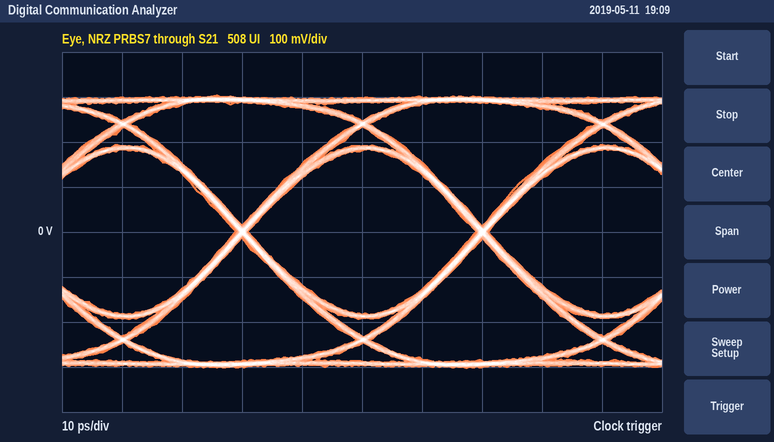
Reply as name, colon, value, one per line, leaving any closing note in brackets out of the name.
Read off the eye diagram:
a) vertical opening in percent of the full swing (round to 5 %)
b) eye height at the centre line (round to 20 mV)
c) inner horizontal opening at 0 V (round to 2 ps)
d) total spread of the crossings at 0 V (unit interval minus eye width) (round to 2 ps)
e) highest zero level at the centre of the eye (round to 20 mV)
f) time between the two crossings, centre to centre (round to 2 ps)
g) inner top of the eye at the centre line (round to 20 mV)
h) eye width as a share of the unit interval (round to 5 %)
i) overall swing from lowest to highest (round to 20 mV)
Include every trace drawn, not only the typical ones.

vertical opening in percent of the full swing: 60 %
eye height at the centre line: 360 mV
inner horizontal opening at 0 V: 38 ps
total spread of the crossings at 0 V (unit interval minus eye width): 2 ps
highest zero level at the centre of the eye: -180 mV
time between the two crossings, centre to centre: 40 ps
inner top of the eye at the centre line: 180 mV
eye width as a share of the unit interval: 95 %
overall swing from lowest to highest: 600 mV
